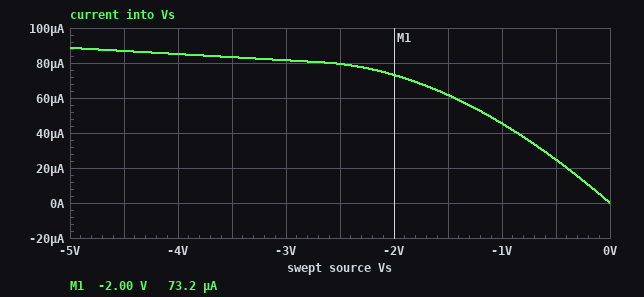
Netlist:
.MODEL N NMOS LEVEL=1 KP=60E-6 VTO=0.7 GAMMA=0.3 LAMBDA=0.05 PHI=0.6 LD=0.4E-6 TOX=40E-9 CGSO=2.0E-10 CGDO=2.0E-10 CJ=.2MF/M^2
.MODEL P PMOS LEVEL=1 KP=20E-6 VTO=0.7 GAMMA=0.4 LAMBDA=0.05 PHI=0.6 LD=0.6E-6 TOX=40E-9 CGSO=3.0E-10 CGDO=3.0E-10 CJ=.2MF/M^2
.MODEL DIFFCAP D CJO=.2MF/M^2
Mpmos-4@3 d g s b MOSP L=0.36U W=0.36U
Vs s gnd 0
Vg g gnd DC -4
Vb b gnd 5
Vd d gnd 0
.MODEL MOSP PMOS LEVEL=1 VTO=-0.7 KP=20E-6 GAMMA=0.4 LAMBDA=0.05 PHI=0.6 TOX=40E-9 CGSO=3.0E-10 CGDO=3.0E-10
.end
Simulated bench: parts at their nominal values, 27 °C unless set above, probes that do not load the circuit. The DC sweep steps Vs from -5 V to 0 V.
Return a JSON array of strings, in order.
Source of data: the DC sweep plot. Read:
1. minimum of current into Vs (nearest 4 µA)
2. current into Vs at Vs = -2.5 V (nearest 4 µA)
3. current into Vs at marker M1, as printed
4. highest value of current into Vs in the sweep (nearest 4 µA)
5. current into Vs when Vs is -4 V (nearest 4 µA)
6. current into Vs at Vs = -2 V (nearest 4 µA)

["0 A", "80 µA", "73.2 µA", "88 µA", "84 µA", "72 µA"]
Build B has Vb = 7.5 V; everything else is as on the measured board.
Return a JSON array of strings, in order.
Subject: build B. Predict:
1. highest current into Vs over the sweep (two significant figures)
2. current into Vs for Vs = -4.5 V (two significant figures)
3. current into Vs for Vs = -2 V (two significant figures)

["76 µA", "75 µA", "65 µA"]
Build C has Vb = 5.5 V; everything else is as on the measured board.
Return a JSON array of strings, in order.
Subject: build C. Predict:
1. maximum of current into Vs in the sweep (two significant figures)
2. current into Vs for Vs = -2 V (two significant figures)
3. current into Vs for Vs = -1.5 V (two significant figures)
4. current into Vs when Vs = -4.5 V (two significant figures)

["86 µA", "71 µA", "60 µA", "84 µA"]
